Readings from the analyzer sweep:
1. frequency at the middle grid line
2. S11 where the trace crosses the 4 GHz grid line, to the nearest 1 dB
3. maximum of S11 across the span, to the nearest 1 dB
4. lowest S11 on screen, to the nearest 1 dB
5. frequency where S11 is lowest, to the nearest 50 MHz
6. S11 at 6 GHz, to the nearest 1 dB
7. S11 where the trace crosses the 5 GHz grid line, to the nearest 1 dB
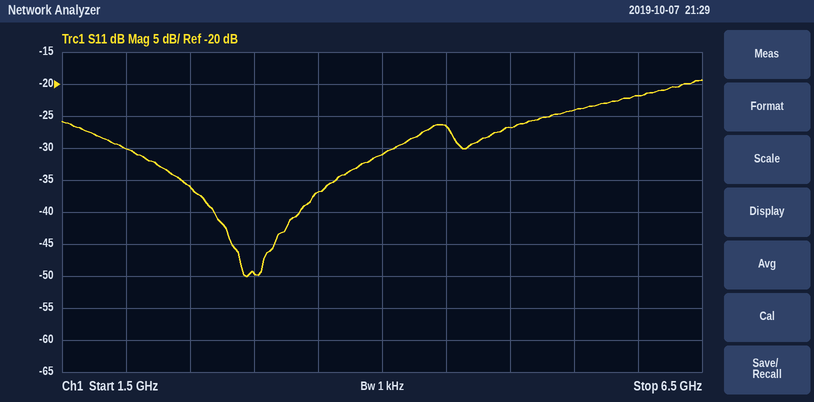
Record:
4 GHz
-31 dB
-19 dB
-50 dB
2.95 GHz
-22 dB
-27 dB
